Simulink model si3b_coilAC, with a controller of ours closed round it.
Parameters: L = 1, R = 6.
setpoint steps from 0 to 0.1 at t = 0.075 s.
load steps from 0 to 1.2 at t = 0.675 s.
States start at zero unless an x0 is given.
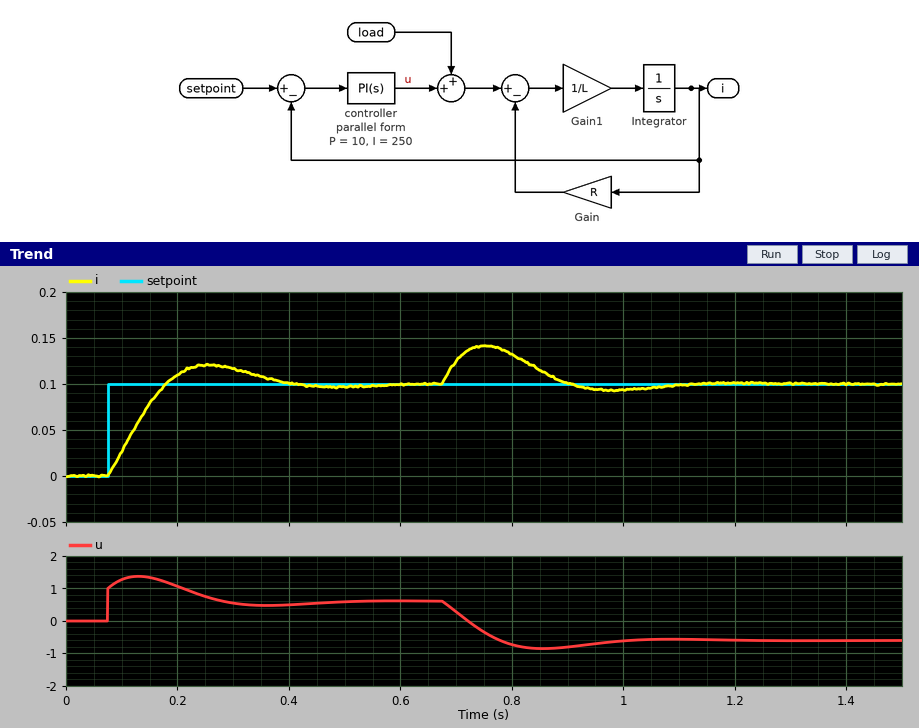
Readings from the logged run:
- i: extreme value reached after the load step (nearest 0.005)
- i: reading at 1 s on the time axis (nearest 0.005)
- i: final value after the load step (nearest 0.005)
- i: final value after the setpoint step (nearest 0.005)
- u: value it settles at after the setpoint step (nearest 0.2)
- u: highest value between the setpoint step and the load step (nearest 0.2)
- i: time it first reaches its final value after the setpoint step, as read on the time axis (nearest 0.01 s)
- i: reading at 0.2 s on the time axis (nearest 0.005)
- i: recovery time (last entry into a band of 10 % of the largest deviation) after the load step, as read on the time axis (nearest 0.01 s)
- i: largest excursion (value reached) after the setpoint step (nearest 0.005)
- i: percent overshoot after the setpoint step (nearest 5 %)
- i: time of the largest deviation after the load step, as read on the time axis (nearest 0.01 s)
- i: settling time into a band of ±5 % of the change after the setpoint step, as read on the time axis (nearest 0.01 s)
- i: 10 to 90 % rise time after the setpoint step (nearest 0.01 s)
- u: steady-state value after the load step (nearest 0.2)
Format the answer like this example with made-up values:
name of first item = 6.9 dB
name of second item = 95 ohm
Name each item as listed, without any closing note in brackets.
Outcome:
i: extreme value reached after the load step = 0.140
i: reading at 1 s on the time axis = 0.095
i: final value after the load step = 0.100
i: final value after the setpoint step = 0.100
u: value it settles at after the setpoint step = 0.6
u: highest value between the setpoint step and the load step = 1.4
i: time it first reaches its final value after the setpoint step, as read on the time axis = 0.18 s
i: reading at 0.2 s on the time axis = 0.110
i: recovery time (last entry into a band of 10 % of the largest deviation) after the load step, as read on the time axis = 1.05 s
i: largest excursion (value reached) after the setpoint step = 0.120
i: percent overshoot after the setpoint step = 20 %
i: time of the largest deviation after the load step, as read on the time axis = 0.75 s
i: settling time into a band of ±5 % of the change after the setpoint step, as read on the time axis = 0.37 s
i: 10 to 90 % rise time after the setpoint step = 0.08 s
u: steady-state value after the load step = -0.6
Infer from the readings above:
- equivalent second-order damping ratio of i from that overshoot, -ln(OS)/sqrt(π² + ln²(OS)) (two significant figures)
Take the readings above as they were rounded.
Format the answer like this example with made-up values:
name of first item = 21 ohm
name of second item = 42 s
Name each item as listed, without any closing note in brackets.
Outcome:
equivalent second-order damping ratio of i from that overshoot, -ln(OS)/sqrt(π² + ln²(OS)) = 0.46
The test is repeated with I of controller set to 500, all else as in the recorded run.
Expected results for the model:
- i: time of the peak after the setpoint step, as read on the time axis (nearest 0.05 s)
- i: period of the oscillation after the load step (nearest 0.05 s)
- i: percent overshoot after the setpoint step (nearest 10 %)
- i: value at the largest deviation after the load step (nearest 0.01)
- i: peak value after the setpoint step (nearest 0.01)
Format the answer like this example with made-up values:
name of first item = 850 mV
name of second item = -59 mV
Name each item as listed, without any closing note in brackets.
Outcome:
i: time of the peak after the setpoint step, as read on the time axis = 0.20 s
i: period of the oscillation after the load step = 0.30 s
i: percent overshoot after the setpoint step = 30 %
i: value at the largest deviation after the load step = 0.13
i: peak value after the setpoint step = 0.13
